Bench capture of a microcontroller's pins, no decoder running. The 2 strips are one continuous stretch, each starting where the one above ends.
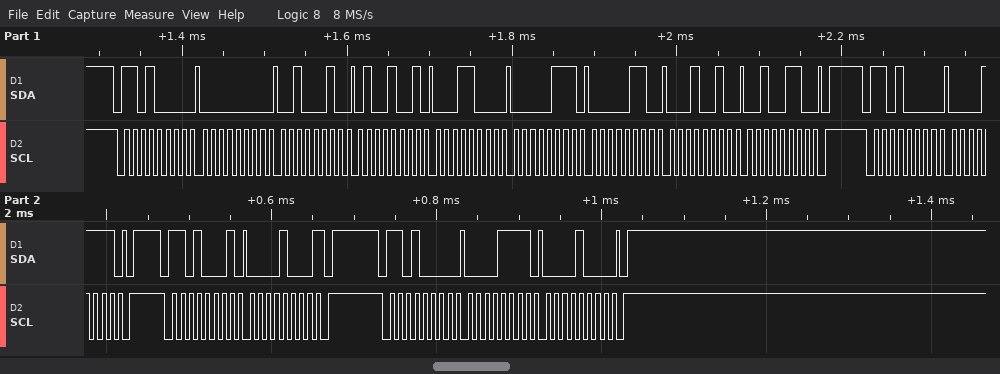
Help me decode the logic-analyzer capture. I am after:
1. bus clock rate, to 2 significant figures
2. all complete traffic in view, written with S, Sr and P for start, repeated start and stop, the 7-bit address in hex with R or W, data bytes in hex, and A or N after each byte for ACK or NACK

100 kHz
S 68W A 00 A 22 A 49 A 18 A 07 A 06 A 12 A 26 A P S 68W A 0F A P S 68R A 08 N P S 68W A 0F A 08 A P
